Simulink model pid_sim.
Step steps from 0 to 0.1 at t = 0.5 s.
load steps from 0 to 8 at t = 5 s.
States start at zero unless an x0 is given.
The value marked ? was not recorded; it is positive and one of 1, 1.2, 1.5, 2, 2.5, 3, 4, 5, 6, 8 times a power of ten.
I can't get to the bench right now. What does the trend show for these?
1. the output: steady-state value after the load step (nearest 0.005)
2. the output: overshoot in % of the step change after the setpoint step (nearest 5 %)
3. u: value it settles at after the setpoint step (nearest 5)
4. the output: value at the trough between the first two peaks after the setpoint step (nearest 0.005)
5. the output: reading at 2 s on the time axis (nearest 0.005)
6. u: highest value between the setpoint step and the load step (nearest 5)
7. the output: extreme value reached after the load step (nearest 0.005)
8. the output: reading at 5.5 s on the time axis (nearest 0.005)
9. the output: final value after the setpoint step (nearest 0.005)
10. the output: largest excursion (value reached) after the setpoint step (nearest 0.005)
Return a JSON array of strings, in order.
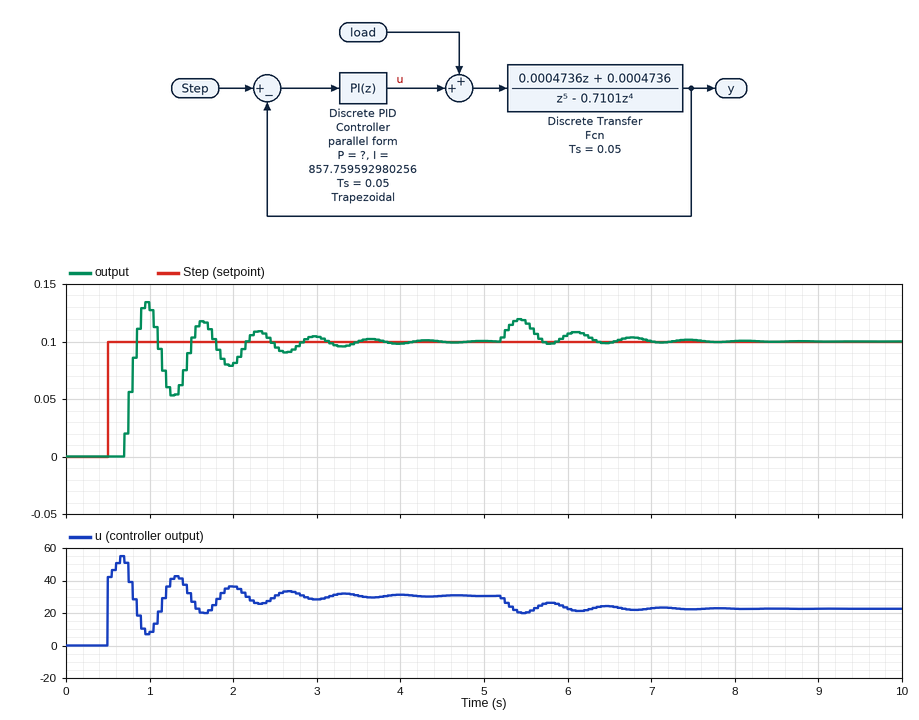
["0.100", "35 %", "30", "0.055", "0.080", "55", "0.120", "0.115", "0.100", "0.135"]
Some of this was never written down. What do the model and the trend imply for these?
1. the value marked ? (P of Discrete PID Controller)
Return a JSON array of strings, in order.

["400"]
